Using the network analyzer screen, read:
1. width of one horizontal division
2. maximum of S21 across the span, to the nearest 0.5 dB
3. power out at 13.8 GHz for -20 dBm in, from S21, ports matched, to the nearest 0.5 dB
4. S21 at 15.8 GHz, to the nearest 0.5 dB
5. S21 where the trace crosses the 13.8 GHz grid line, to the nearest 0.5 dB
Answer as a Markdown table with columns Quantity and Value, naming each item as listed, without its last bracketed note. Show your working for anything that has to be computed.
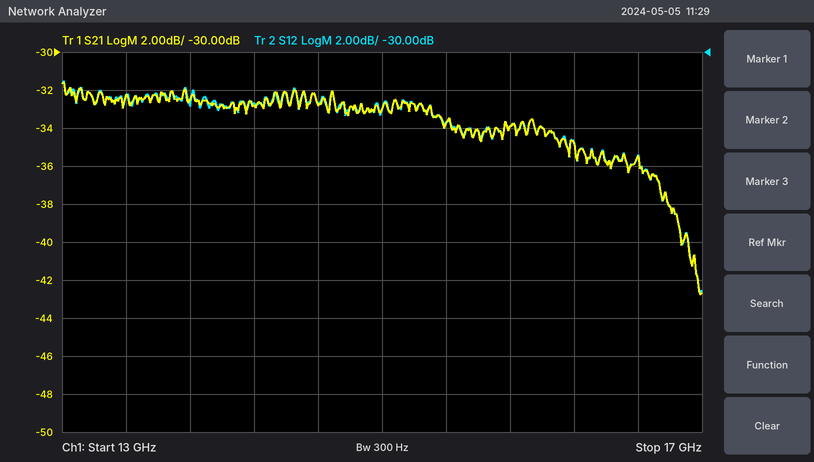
| Quantity | Value |
|---|---|
| width of one horizontal division | 400 MHz |
| maximum of S21 across the span, to the nearest 0.5 dB | -31.5 dB |
| power out at 13.8 GHz for -20 dBm in, from S21, ports matched, to the nearest 0.5 dB | -20 dBm + (-32.5 dB) = -52.5 dBm |
| S21 at 15.8 GHz, to the nearest 0.5 dB | -34.0 dB |
| S21 where the trace crosses the 13.8 GHz grid line, to the nearest 0.5 dB | -32.5 dB |
